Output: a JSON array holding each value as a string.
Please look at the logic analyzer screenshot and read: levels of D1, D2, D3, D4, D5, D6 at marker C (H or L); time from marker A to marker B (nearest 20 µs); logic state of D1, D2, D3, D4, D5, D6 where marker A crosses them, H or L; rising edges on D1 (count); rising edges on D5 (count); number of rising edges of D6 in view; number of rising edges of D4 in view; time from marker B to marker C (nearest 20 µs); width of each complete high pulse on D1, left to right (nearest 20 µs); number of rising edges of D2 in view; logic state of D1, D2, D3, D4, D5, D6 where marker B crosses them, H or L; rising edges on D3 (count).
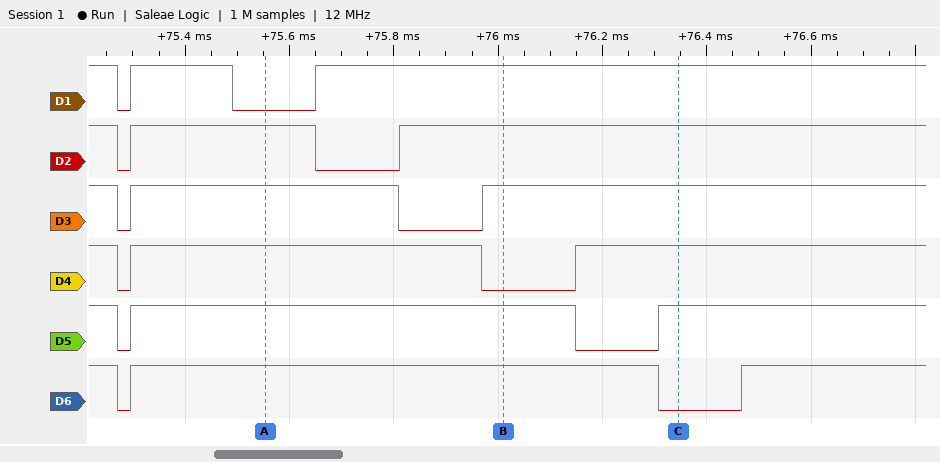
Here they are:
["D1=H, D2=H, D3=H, D4=H, D5=H, D6=L", "460 µs", "D1=L, D2=H, D3=H, D4=H, D5=H, D6=H", "2", "2", "2", "2", "340 µs", "200 µs", "2", "D1=H, D2=H, D3=H, D4=L, D5=H, D6=H", "2"]
